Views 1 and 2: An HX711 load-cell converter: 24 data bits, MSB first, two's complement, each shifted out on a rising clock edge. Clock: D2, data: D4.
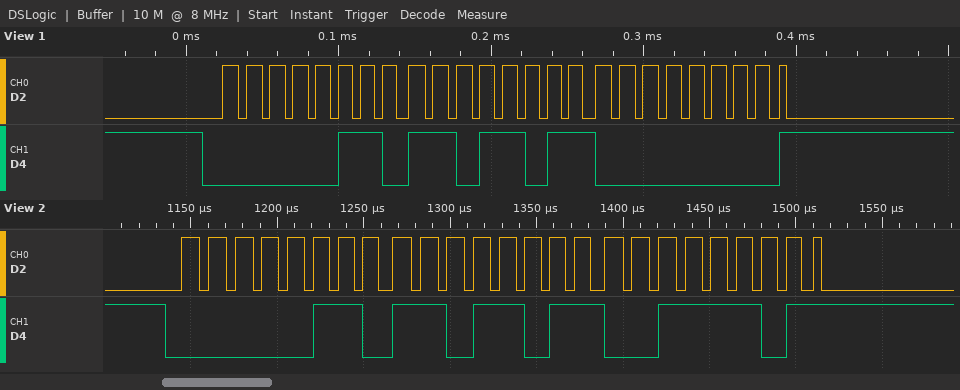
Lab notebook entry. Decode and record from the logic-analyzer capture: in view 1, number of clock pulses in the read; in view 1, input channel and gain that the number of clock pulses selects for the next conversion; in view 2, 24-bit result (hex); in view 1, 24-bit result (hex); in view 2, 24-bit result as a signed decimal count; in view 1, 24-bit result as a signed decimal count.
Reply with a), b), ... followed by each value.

a) 25
b) channel A, gain 128
c) 0x06DB3D
d) 0x06DB00
e) 449341
f) 449280
